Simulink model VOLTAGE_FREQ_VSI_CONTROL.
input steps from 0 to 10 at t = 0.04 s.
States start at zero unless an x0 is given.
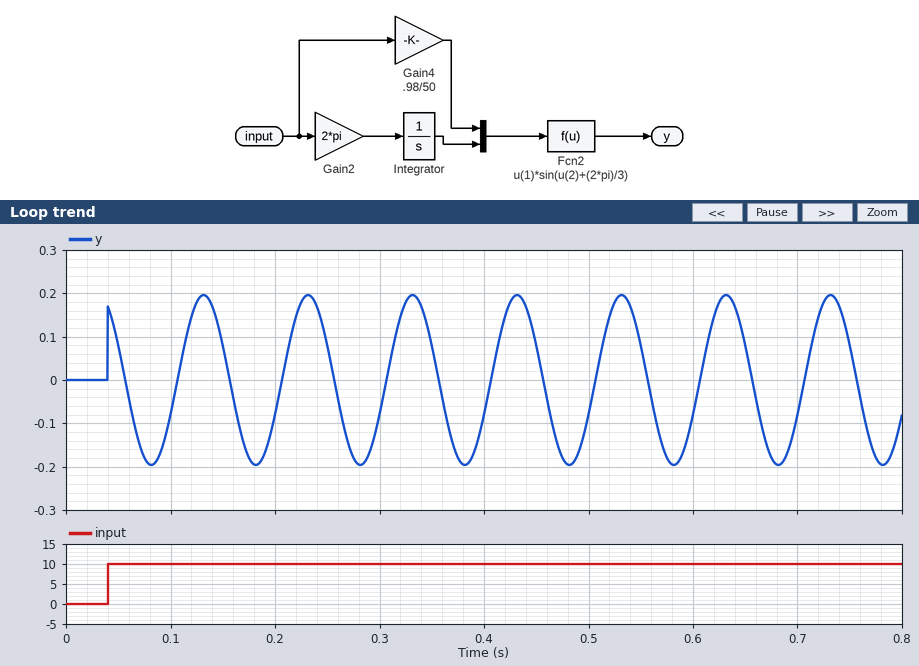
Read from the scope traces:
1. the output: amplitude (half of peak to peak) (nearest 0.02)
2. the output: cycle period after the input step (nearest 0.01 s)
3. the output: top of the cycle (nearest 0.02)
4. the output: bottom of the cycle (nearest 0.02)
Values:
0.20
0.10 s
0.20
-0.20
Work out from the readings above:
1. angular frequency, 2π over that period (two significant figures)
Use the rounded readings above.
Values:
63 rad/s
